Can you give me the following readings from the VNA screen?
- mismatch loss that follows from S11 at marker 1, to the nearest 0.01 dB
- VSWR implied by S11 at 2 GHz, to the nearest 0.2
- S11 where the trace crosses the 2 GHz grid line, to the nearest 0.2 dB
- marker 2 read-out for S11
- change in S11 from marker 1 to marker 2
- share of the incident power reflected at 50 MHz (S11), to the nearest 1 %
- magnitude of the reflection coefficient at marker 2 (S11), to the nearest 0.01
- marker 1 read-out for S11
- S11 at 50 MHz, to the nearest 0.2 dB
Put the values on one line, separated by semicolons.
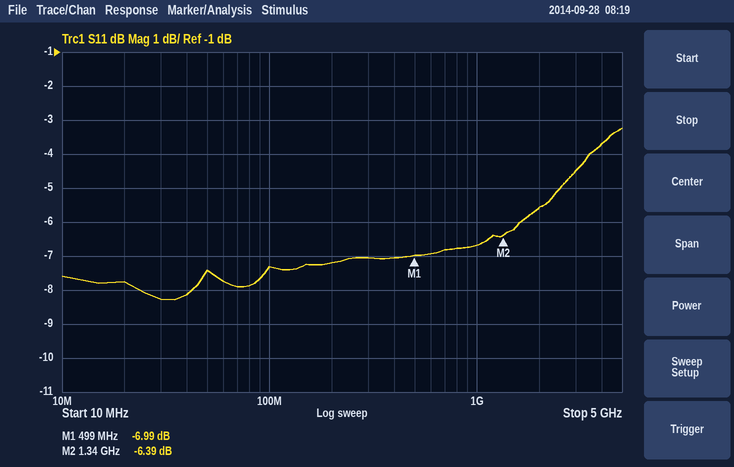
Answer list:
0.97 dB; 3.2; -5.6 dB; -6.39 dB; 0.60 dB; 18 %; 0.48; -6.99 dB; -7.4 dB
